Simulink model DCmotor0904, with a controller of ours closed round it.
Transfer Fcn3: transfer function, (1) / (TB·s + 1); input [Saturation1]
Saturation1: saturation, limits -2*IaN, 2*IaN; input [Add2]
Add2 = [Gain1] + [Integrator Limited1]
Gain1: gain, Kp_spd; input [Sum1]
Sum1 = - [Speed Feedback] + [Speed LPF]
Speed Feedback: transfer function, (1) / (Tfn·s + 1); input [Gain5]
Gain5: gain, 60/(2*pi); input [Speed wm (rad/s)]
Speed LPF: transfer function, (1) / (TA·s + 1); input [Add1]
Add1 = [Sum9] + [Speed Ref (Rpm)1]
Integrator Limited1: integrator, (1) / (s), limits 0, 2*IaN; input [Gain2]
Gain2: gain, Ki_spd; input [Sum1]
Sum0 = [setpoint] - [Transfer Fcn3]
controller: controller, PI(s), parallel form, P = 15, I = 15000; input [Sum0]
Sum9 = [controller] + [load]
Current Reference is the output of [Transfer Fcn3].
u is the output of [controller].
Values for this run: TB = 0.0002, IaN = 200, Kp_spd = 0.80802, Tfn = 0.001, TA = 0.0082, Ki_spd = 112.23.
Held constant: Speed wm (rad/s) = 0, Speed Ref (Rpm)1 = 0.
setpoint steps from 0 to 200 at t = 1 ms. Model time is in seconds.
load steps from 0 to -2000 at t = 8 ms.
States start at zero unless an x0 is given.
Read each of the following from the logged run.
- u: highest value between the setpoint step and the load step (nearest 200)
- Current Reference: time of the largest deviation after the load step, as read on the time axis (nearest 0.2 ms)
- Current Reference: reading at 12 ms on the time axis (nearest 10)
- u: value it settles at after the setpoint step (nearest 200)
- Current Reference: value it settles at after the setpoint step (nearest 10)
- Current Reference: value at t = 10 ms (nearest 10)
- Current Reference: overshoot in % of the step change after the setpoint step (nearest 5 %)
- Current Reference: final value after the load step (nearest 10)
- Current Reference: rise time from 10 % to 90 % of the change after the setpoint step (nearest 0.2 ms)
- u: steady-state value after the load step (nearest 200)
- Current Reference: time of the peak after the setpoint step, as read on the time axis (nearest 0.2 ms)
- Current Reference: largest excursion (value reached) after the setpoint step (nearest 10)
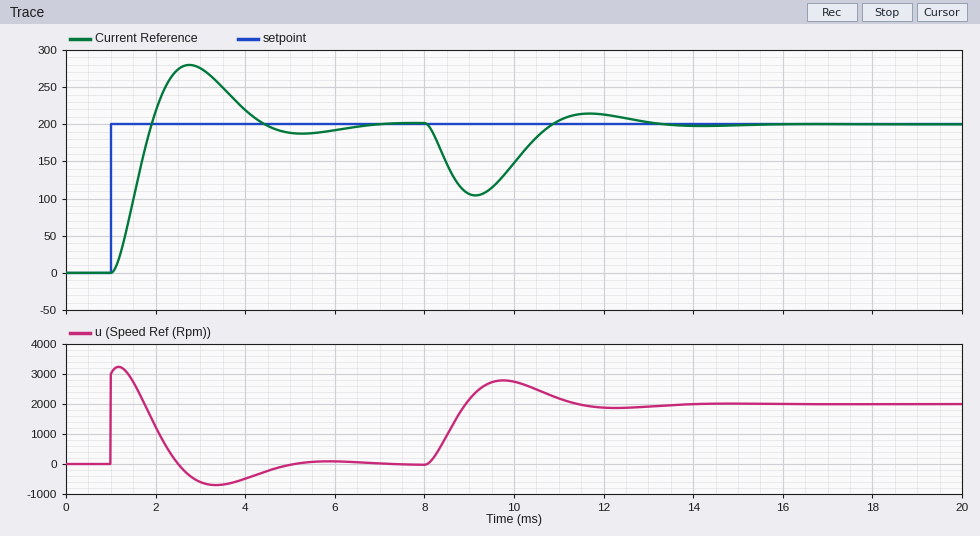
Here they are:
3200
9.2 ms
210
0
200
150
40 %
200
0.6 ms
2000
2.8 ms
280
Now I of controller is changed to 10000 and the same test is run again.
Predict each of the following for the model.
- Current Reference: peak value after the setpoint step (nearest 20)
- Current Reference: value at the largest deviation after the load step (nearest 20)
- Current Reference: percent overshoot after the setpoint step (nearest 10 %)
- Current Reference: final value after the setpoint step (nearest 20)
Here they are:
260
100
30 %
200
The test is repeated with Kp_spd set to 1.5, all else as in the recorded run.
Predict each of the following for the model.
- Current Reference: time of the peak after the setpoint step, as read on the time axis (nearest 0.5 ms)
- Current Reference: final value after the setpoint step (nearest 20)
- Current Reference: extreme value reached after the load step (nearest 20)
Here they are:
2.0 ms
200
80
